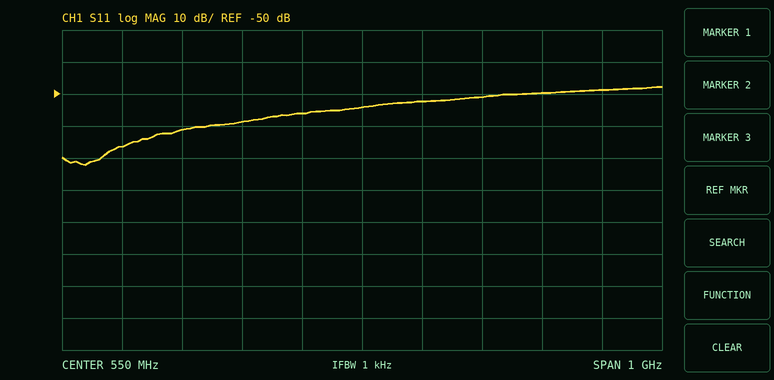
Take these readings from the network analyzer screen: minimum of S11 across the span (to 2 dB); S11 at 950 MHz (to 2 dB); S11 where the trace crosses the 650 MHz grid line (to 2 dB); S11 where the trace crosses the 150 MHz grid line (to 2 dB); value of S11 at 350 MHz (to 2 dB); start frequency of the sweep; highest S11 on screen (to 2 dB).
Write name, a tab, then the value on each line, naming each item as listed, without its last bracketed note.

minimum of S11 across the span	-72 dB
S11 at 950 MHz	-48 dB
S11 where the trace crosses the 650 MHz grid line	-52 dB
S11 where the trace crosses the 150 MHz grid line	-66 dB
value of S11 at 350 MHz	-58 dB
start frequency of the sweep	50 MHz
highest S11 on screen	-48 dB
